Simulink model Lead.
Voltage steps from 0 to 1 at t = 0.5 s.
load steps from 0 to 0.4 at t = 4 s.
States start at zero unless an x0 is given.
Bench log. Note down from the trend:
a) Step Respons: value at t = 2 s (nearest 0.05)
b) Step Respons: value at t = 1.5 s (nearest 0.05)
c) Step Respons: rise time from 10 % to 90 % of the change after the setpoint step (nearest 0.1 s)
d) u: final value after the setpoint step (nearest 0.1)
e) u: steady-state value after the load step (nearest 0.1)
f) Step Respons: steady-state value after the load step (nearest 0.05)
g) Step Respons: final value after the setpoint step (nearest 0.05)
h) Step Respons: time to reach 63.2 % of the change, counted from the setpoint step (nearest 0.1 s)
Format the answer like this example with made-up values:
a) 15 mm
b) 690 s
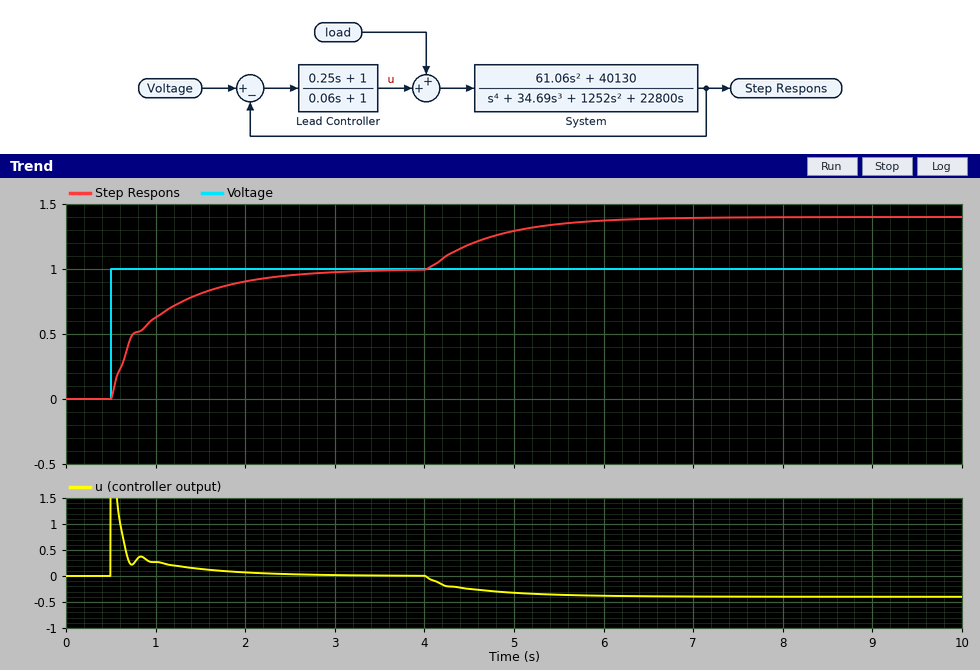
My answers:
a) 0.90
b) 0.80
c) 1.4 s
d) 0.0
e) -0.4
f) 1.40
g) 1.00
h) 0.5 s
